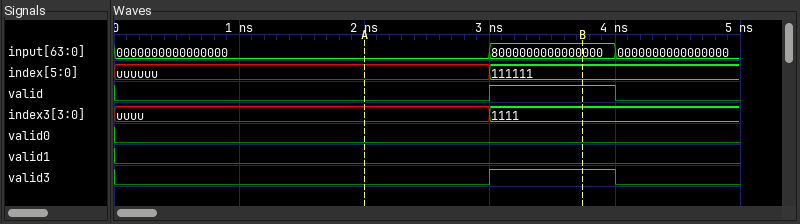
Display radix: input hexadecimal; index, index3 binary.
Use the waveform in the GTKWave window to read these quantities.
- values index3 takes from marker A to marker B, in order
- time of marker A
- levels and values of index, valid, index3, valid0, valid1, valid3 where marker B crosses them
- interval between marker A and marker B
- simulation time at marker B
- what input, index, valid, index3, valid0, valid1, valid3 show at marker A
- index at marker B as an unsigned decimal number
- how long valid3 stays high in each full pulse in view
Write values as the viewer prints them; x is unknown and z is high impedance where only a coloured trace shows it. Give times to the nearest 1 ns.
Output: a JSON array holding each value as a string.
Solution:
["uuuu, 1111", "2 ns", "index=111111, valid=1, index3=1111, valid0=0, valid1=0, valid3=1", "2 ns", "4 ns", "input=0000000000000000, index=uuuuuu, valid=0, index3=uuuu, valid0=0, valid1=0, valid3=0", "63", "1 ns"]
